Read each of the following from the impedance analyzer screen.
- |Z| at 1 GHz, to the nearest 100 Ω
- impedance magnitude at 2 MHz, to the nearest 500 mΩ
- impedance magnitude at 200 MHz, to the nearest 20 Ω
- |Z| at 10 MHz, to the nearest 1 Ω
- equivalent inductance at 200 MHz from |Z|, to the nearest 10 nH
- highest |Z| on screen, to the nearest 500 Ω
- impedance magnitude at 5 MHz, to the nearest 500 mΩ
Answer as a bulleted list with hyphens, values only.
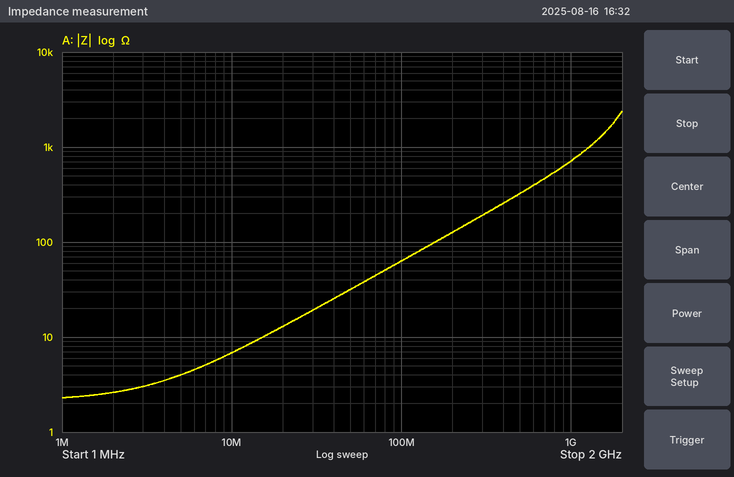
- 700 Ω
- 2.5 Ω
- 120 Ω
- 7 Ω
- 100 nH
- 2.5 kΩ
- 4.0 Ω
